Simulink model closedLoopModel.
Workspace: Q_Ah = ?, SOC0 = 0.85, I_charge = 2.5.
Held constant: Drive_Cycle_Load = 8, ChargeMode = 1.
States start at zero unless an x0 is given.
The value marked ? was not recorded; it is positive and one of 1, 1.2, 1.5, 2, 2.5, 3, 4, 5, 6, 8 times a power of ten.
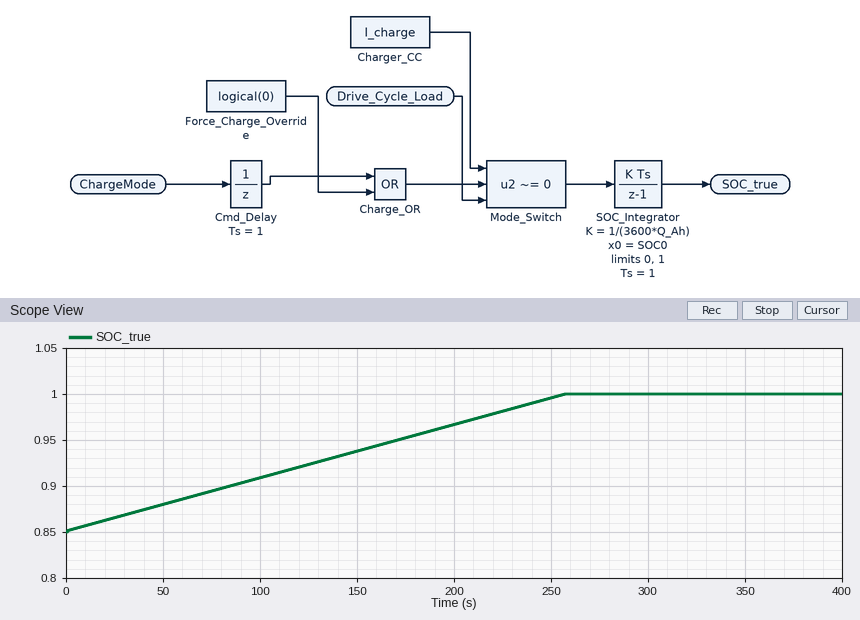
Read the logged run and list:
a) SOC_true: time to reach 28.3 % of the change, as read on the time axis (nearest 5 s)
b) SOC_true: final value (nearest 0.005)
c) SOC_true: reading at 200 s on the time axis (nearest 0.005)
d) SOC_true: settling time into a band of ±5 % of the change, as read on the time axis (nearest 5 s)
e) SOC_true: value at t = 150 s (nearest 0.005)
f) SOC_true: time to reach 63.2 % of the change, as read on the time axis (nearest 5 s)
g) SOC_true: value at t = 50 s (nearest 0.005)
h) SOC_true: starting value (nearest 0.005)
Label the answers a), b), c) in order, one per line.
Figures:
a) 70 s
b) 1.000
c) 0.965
d) 245 s
e) 0.940
f) 160 s
g) 0.880
h) 0.850
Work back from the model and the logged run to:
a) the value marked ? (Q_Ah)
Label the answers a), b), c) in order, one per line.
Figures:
a) 1.2
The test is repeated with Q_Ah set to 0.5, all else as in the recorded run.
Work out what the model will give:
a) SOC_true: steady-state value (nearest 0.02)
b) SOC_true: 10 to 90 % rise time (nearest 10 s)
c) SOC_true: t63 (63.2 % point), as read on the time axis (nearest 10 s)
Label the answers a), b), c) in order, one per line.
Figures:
a) 1.00
b) 90 s
c) 70 s
